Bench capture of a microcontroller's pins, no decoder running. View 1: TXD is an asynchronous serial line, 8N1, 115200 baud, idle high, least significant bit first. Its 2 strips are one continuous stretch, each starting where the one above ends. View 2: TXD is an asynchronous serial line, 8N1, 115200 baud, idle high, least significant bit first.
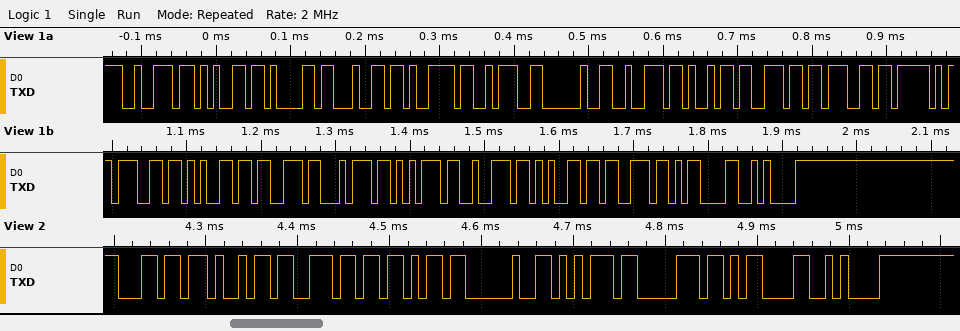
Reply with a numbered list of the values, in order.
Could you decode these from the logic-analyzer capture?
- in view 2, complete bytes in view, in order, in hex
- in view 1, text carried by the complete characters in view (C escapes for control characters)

1. 0x6C 0x69 0x6E 0x6B 0x20 0x75 0x70 0x0D 0x0A
2. "ready: ring_gestures\r\n"
